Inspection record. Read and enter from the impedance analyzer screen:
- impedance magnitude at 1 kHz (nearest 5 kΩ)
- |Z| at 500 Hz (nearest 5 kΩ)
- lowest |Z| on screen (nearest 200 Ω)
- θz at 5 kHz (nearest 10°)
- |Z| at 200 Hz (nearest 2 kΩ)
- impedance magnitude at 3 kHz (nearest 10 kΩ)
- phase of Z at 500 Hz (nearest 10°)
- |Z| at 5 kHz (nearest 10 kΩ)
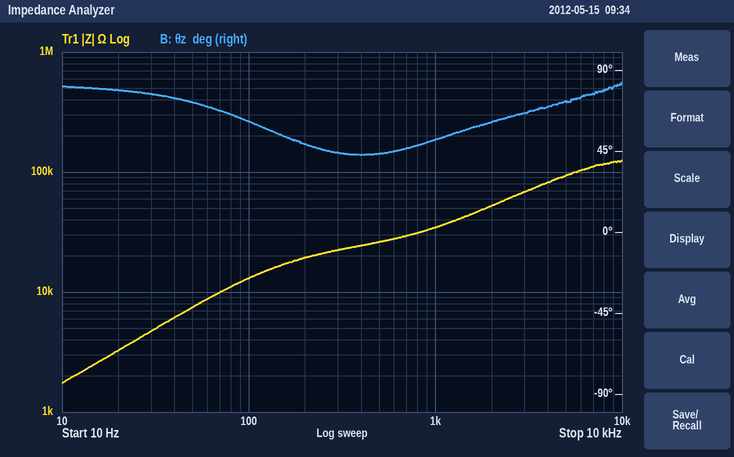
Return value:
35 kΩ
25 kΩ
1.8 kΩ
70°
20 kΩ
70 kΩ
40°
90 kΩ
